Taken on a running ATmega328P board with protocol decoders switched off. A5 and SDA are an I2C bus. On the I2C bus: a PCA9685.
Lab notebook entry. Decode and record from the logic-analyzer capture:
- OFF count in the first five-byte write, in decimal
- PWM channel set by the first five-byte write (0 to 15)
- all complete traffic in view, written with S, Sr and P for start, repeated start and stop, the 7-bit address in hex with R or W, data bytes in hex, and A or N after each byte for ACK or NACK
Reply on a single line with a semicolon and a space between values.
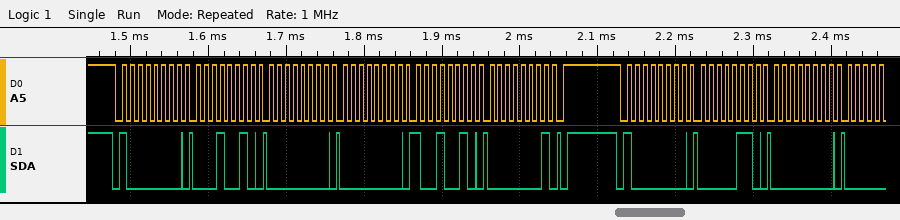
402; 3; S 40W A 12 A 00 A 00 A 92 A 01 A P S 40W A 06 A 00 A
